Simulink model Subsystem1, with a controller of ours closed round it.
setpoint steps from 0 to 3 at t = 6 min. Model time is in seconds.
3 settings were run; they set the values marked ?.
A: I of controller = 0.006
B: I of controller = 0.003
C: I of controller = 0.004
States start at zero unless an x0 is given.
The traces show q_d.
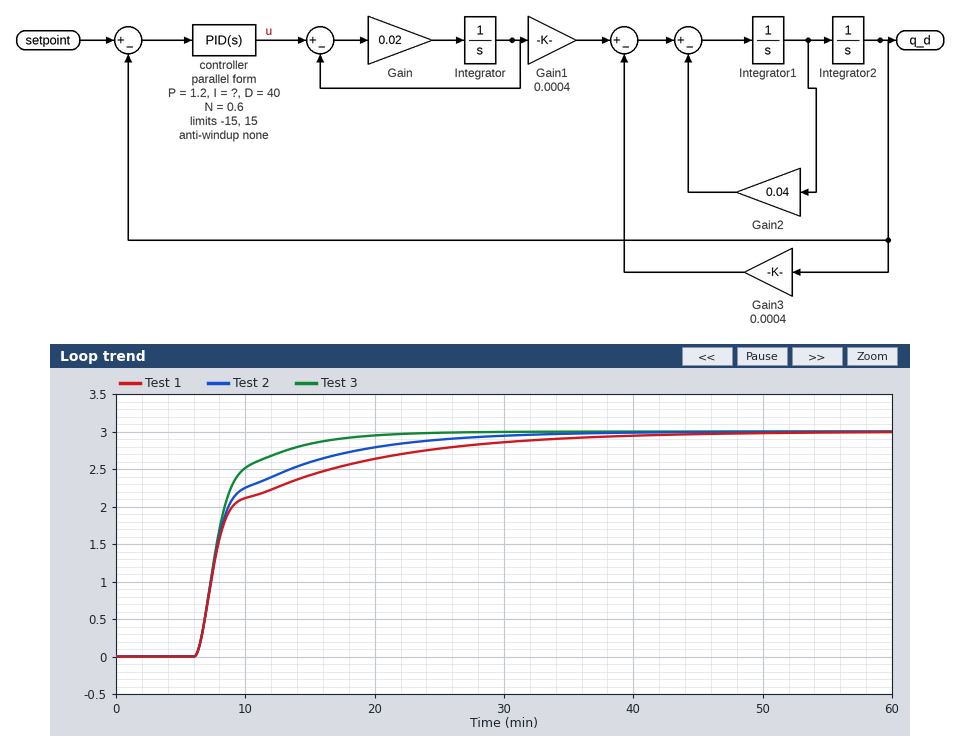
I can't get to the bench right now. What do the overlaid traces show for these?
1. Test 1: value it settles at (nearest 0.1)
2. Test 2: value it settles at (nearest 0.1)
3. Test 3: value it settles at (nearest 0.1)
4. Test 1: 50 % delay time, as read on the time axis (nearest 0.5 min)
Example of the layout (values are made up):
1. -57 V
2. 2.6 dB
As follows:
1. 3.0
2. 3.0
3. 3.0
4. 8.0 min
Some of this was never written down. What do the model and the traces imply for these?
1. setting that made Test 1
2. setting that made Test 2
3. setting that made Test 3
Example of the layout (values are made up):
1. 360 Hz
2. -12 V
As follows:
1. B
2. C
3. A
